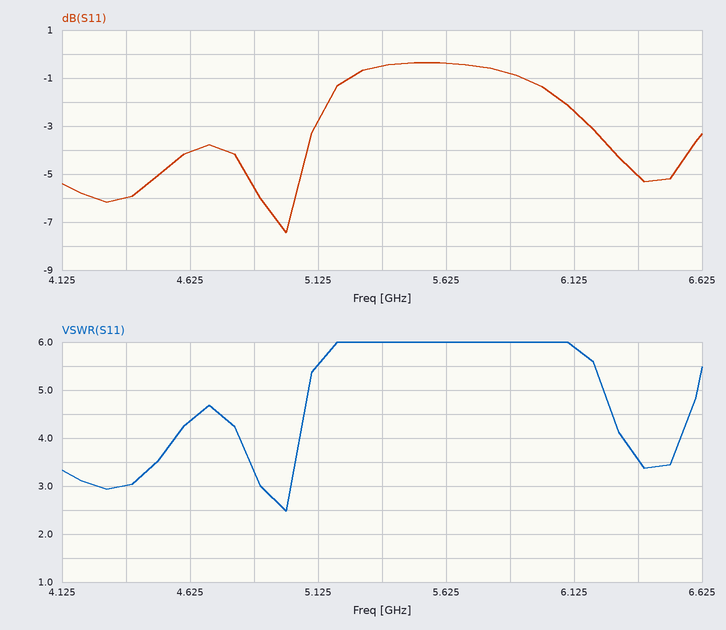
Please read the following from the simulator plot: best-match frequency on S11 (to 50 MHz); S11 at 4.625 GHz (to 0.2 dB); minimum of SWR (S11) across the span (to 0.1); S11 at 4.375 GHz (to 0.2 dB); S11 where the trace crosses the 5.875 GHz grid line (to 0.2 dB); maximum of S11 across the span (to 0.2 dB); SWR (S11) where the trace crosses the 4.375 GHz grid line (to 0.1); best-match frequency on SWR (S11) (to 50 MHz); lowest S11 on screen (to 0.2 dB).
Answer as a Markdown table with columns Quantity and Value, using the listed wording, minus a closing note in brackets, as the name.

| Quantity | Value |
|---|---|
| best-match frequency on S11 | 5.00 GHz |
| S11 at 4.625 GHz | -4.0 dB |
| minimum of SWR (S11) across the span | 2.5 |
| S11 at 4.375 GHz | -6.0 dB |
| S11 where the trace crosses the 5.875 GHz grid line | -0.8 dB |
| maximum of S11 across the span | -0.4 dB |
| SWR (S11) where the trace crosses the 4.375 GHz grid line | 3.0 |
| best-match frequency on SWR (S11) | 5.00 GHz |
| lowest S11 on screen | -7.4 dB |
